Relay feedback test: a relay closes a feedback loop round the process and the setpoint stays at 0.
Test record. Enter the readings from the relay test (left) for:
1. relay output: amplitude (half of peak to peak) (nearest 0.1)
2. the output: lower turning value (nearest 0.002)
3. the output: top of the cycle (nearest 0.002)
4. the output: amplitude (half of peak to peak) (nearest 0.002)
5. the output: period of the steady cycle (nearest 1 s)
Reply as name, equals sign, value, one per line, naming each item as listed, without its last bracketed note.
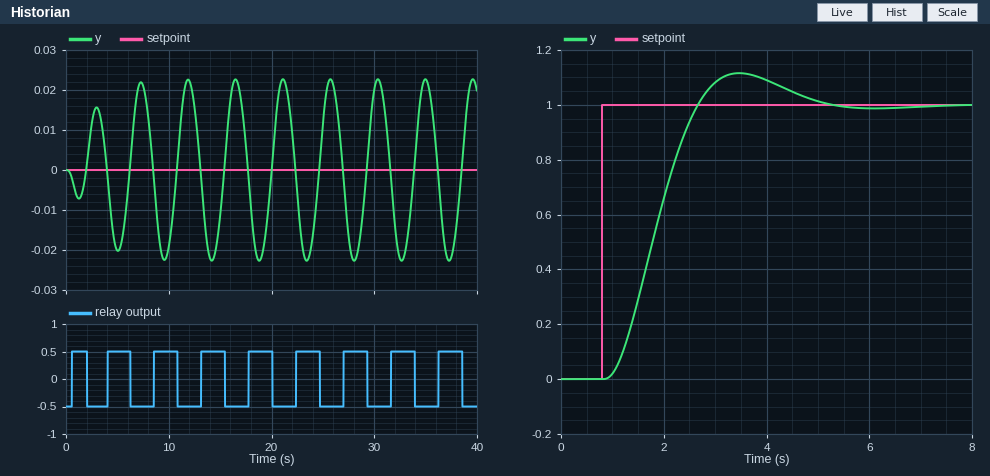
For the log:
relay output: amplitude (half of peak to peak) = 0.5
the output: lower turning value = -0.022
the output: top of the cycle = 0.022
the output: amplitude (half of peak to peak) = 0.022
the output: period of the steady cycle = 5 s
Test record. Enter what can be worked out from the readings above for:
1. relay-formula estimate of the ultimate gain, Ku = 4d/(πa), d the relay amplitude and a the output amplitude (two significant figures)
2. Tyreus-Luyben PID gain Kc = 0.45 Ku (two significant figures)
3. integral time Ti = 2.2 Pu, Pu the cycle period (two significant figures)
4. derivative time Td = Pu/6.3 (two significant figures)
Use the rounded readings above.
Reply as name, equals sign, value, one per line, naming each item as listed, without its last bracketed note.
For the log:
relay-formula estimate of the ultimate gain, Ku = 4d/(πa), d the relay amplitude and a the output amplitude = 29
Tyreus-Luyben PID gain Kc = 0.45 Ku = 13
integral time Ti = 2.2 Pu, Pu the cycle period = 11 s
derivative time Td = Pu/6.3 = 0.79 s
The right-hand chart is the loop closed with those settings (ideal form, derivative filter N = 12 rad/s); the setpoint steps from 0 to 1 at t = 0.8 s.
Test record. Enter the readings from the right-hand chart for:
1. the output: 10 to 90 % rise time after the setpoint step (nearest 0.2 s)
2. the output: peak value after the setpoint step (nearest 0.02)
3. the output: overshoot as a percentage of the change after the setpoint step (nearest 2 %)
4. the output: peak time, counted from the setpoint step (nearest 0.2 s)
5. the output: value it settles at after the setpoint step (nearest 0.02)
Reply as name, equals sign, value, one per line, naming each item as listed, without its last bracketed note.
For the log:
the output: 10 to 90 % rise time after the setpoint step = 1.2 s
the output: peak value after the setpoint step = 1.12
the output: overshoot as a percentage of the change after the setpoint step = 12 %
the output: peak time, counted from the setpoint step = 2.6 s
the output: value it settles at after the setpoint step = 1.00
